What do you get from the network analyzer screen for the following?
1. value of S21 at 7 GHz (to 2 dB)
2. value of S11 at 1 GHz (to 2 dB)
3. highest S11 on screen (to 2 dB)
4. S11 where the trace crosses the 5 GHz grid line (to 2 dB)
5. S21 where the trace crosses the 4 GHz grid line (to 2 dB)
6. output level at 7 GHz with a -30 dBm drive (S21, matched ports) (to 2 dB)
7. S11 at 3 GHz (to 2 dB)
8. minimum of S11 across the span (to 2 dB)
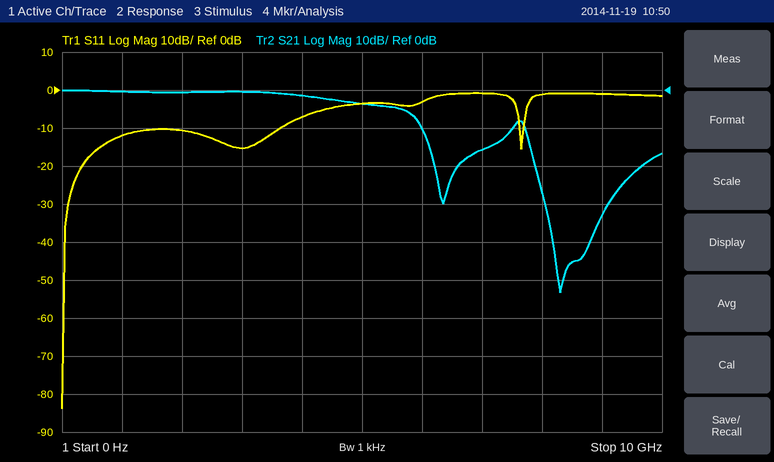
-16 dB
-12 dB
0 dB
-4 dB
-2 dB
-46 dBm
-16 dB
-84 dB
